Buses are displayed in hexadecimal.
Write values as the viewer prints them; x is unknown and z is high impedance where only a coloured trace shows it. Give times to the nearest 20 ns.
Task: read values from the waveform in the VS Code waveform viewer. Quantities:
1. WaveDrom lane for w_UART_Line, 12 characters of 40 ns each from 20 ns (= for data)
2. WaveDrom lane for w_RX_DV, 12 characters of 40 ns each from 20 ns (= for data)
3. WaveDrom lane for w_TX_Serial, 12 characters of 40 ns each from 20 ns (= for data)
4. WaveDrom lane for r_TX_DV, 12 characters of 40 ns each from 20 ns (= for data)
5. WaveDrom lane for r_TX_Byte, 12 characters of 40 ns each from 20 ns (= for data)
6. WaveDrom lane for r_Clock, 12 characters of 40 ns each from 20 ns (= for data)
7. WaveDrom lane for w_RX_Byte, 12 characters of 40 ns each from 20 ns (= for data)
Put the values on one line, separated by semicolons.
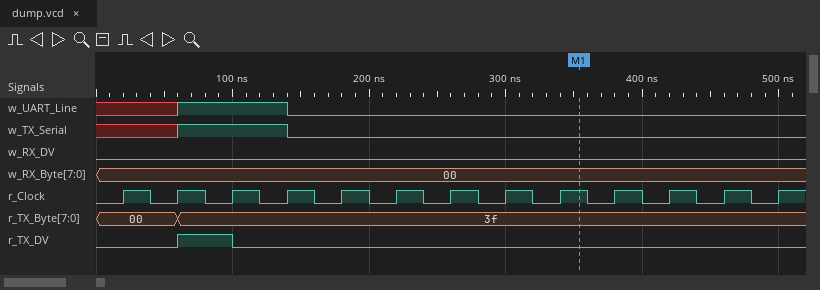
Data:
{name: 'w_UART_Line', wave: 'x1.0........'}; {name: 'w_RX_DV', wave: '0...........'}; {name: 'w_TX_Serial', wave: 'x1.0........'}; {name: 'r_TX_DV', wave: '010.........'}; {name: 'r_TX_Byte', wave: '==..........', data: '00 3f'}; {name: 'r_Clock', wave: 'p...........'}; {name: 'w_RX_Byte', wave: '=...........', data: '00'}
